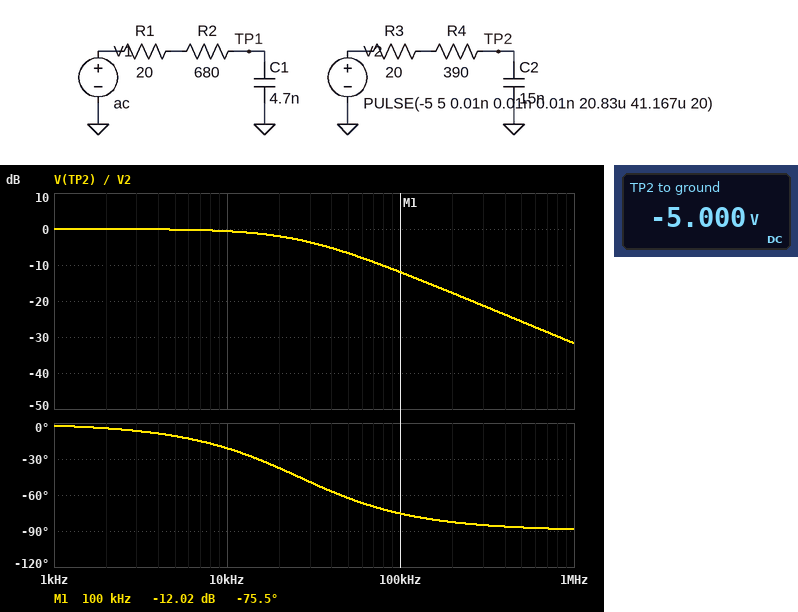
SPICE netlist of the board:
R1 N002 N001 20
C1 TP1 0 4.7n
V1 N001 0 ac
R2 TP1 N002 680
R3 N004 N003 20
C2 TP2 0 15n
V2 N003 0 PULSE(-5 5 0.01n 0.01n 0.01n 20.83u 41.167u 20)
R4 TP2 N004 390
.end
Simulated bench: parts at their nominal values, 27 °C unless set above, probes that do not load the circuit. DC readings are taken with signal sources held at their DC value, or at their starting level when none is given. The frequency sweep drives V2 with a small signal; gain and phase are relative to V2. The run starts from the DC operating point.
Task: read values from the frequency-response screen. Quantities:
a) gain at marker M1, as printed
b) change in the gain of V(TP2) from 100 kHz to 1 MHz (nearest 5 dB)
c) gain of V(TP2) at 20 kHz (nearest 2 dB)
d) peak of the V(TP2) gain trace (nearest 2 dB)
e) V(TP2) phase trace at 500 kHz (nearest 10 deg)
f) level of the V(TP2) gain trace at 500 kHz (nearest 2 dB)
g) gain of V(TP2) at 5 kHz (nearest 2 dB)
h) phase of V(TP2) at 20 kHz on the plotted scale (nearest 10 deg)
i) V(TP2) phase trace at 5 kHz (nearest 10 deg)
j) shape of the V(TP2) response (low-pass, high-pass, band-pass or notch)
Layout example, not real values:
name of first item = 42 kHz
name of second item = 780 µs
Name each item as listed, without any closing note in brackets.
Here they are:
gain at marker M1, as printed = -12.02 dB
change in the gain of V(TP2) from 100 kHz to 1 MHz = -20 dB
gain of V(TP2) at 20 kHz = -2 dB
peak of the V(TP2) gain trace = 0 dB
V(TP2) phase trace at 500 kHz = -90 deg
level of the V(TP2) gain trace at 500 kHz = -26 dB
gain of V(TP2) at 5 kHz = 0 dB
phase of V(TP2) at 20 kHz on the plotted scale = -40 deg
V(TP2) phase trace at 5 kHz = -10 deg
shape of the V(TP2) response = low-pass
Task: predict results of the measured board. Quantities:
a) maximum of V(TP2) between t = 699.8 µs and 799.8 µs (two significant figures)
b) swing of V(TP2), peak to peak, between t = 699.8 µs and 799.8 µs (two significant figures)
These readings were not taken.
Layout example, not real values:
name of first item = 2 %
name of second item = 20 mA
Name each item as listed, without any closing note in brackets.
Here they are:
maximum of V(TP2) between t = 699.8 µs and 799.8 µs = 4.7 V
swing of V(TP2), peak to peak, between t = 699.8 µs and 799.8 µs = 9.3 V
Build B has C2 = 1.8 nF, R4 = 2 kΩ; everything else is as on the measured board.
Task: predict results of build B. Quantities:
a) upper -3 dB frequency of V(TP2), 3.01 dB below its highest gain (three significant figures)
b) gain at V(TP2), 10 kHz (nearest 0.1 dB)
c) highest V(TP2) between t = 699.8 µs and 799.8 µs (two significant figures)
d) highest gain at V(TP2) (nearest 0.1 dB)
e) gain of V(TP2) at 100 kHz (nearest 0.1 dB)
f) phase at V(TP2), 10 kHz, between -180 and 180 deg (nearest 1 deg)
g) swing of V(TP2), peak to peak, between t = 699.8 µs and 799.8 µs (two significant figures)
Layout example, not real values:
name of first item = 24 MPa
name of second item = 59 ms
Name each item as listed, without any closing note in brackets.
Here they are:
upper -3 dB frequency of V(TP2), 3.01 dB below its highest gain = 43.8 kHz
gain at V(TP2), 10 kHz = -0.2 dB
highest V(TP2) between t = 699.8 µs and 799.8 µs = 5.0 V
highest gain at V(TP2) = 0 dB
gain of V(TP2) at 100 kHz = -7.9 dB
phase at V(TP2), 10 kHz, between -180 and 180 deg = -13 deg
swing of V(TP2), peak to peak, between t = 699.8 µs and 799.8 µs = 9.9 V
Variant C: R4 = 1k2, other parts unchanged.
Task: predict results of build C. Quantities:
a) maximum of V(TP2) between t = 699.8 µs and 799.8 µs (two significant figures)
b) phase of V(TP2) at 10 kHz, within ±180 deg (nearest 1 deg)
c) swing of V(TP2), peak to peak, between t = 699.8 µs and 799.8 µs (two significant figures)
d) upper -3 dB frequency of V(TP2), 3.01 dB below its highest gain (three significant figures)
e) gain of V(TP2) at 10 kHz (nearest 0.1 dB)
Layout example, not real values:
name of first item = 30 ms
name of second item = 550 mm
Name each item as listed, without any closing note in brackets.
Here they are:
maximum of V(TP2) between t = 699.8 µs and 799.8 µs = 2.6 V
phase of V(TP2) at 10 kHz, within ±180 deg = -49 deg
swing of V(TP2), peak to peak, between t = 699.8 µs and 799.8 µs = 5.1 V
upper -3 dB frequency of V(TP2), 3.01 dB below its highest gain = 8.70 kHz
gain of V(TP2) at 10 kHz = -3.7 dB
